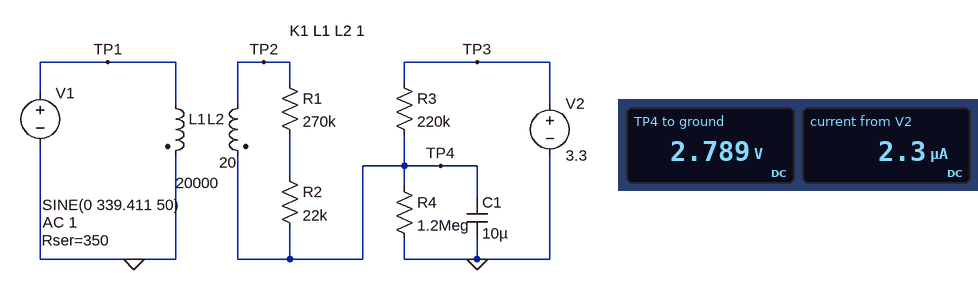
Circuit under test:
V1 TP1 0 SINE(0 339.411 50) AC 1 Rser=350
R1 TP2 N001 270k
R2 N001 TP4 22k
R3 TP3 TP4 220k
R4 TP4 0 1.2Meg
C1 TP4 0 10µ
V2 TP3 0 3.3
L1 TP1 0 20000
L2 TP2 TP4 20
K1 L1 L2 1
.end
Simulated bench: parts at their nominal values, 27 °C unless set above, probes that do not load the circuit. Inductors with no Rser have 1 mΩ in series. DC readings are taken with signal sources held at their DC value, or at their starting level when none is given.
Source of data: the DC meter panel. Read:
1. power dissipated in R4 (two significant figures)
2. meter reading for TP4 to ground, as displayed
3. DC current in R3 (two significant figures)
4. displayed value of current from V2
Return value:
6.5 µW
2.789 V
2.3 µA
2.3 µA
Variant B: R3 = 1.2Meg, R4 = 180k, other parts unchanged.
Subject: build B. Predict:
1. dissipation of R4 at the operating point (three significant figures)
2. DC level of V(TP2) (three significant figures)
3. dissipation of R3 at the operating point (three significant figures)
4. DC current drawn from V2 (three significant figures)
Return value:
1.03 µW
430 mV
6.86 µW
2.39 µA
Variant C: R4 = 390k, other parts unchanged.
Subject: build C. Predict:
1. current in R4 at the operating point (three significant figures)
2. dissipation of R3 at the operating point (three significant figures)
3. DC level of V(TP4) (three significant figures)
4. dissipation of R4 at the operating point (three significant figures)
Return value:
5.41 µA
6.44 µW
2.11 V
11.4 µW
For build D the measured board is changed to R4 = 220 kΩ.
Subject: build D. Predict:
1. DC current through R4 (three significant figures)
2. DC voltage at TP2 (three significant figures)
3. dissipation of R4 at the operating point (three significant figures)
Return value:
7.50 µA
1.65 V
12.4 µW
